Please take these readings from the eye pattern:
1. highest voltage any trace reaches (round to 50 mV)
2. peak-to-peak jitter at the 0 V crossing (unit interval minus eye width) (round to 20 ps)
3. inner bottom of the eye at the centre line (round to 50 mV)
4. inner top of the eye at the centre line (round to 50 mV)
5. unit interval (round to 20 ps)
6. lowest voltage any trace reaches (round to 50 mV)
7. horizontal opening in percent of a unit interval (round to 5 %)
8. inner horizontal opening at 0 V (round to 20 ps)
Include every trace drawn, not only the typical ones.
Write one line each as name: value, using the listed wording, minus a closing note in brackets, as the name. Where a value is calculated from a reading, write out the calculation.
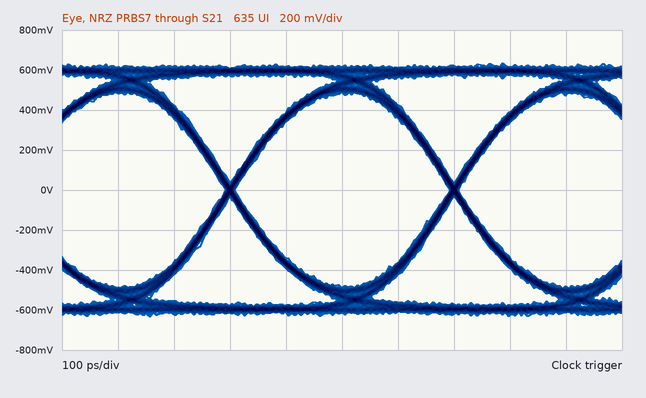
highest voltage any trace reaches: 650 mV
peak-to-peak jitter at the 0 V crossing (unit interval minus eye width): 20 ps
inner bottom of the eye at the centre line: -500 mV
inner top of the eye at the centre line: 500 mV
unit interval: 400 ps
lowest voltage any trace reaches: -650 mV
horizontal opening in percent of a unit interval: 380 ps / 400 ps ≈ 95 %
inner horizontal opening at 0 V: 380 ps
